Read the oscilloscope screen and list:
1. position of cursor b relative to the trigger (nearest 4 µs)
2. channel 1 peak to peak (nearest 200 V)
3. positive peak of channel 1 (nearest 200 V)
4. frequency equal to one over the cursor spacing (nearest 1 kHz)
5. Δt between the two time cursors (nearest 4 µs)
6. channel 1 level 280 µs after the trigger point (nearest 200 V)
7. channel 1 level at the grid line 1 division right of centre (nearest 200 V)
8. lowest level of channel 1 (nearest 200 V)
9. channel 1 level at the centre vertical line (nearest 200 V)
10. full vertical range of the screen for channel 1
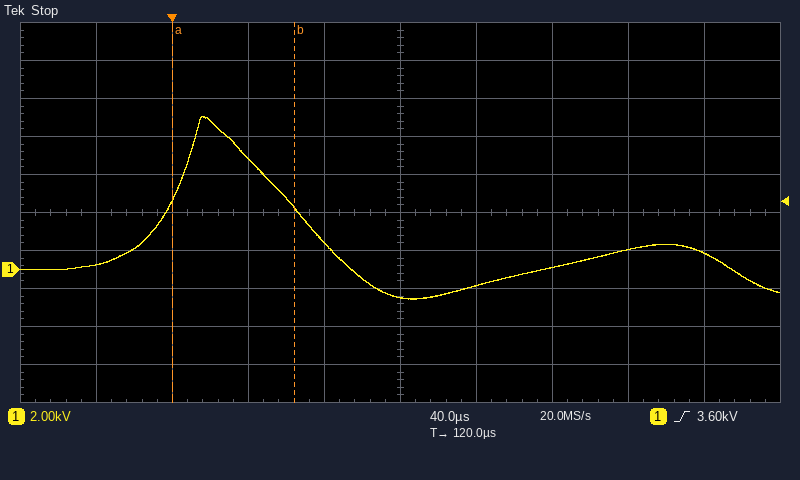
+64 µs
9.6 kV
8.0 kV
16 kHz
64 µs
800 V
-800 V
-1.6 kV
-1.4 kV
20 kV
